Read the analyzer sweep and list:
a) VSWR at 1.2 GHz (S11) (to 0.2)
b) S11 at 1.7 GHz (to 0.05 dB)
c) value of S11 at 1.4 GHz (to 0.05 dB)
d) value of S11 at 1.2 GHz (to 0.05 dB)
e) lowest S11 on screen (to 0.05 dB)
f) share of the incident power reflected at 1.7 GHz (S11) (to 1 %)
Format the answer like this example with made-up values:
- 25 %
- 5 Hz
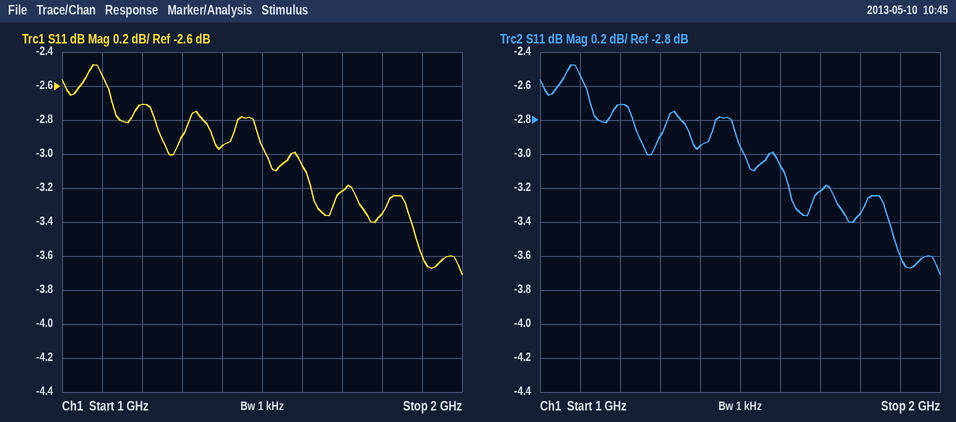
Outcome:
- 6.4
- -3.20 dB
- -2.95 dB
- -2.70 dB
- -3.70 dB
- 48 %
